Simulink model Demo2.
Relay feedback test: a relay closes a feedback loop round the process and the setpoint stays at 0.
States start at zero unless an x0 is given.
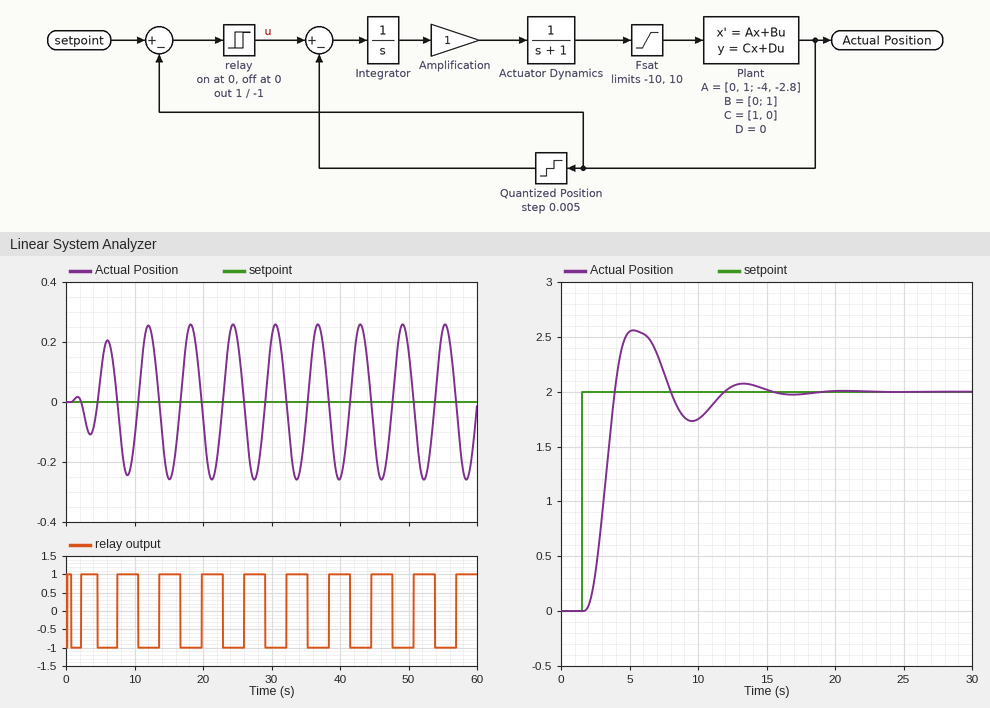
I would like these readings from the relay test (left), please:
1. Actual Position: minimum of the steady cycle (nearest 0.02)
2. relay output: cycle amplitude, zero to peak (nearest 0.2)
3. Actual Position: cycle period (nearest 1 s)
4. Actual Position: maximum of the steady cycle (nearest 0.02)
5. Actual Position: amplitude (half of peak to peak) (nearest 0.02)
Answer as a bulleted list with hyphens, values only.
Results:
- -0.26
- 1.0
- 6 s
- 0.26
- 0.26
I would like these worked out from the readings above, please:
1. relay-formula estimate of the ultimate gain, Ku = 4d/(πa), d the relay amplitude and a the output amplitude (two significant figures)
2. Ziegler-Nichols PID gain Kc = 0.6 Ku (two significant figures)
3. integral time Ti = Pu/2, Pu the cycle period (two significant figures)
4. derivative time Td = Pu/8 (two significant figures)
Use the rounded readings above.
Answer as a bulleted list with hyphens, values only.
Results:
- 4.9
- 2.9
- 3.0 s
- 0.75 s
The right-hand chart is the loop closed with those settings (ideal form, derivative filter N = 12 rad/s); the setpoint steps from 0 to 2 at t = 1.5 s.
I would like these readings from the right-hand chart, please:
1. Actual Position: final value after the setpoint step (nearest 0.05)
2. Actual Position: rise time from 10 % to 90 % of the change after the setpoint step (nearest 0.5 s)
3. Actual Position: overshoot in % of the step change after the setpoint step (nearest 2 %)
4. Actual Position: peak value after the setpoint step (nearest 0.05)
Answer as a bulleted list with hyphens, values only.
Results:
- 2.00
- 1.5 s
- 28 %
- 2.55
